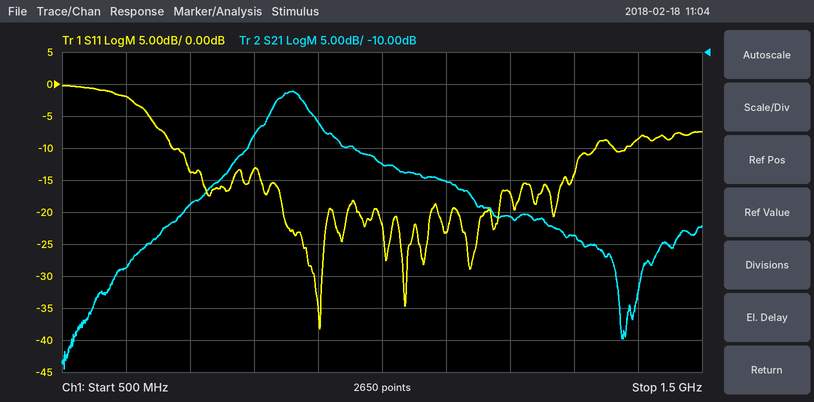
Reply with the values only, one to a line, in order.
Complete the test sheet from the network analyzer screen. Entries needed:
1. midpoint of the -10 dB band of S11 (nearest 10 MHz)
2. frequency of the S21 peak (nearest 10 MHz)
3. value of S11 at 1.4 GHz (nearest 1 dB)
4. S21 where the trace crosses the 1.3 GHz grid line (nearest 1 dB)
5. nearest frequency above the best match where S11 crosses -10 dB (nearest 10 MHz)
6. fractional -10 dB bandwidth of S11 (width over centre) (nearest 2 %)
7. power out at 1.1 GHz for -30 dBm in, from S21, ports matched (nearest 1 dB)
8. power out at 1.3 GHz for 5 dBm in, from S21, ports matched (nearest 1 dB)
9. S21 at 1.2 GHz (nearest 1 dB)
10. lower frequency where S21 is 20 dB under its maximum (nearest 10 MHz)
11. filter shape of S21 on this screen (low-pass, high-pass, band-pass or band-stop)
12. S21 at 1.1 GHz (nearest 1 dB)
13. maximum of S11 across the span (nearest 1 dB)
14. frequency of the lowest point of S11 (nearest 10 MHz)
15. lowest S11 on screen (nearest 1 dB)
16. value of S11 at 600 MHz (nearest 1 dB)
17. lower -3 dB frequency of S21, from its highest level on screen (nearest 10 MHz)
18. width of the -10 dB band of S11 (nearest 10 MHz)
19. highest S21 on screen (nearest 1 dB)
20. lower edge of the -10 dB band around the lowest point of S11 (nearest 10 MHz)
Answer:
1.00 GHz
860 MHz
-9 dB
-39 dB
1.33 GHz
66 %
-60 dBm
-34 dBm
-36 dB
680 MHz
band-pass
-30 dB
0 dB
900 MHz
-38 dB
-2 dB
830 MHz
660 MHz
-16 dB
670 MHz
